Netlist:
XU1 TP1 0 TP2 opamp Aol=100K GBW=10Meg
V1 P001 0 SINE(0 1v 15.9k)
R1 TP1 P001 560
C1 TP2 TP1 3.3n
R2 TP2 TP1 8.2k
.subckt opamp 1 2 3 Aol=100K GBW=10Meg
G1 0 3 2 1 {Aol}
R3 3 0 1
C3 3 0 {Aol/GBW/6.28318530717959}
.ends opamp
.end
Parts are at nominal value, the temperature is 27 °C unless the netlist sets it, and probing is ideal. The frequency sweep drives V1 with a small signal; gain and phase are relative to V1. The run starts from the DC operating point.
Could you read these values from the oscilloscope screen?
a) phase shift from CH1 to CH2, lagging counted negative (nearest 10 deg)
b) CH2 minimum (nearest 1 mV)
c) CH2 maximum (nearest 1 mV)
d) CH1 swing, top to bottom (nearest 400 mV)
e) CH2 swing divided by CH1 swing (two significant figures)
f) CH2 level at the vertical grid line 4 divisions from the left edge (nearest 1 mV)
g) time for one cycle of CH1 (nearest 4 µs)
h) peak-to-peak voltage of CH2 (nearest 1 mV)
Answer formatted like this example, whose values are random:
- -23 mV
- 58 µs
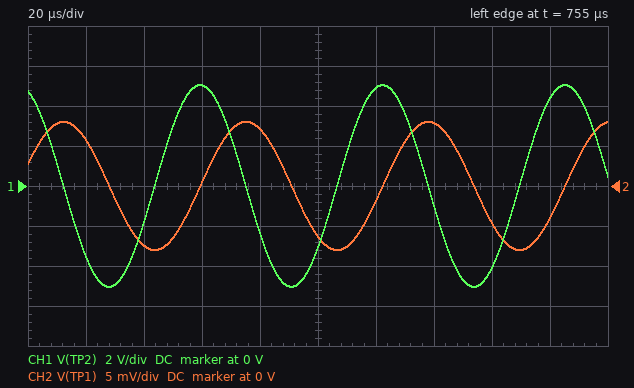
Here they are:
- -90 deg
- -8 mV
- 8 mV
- 10.0 V
- 0.0016
- 7 mV
- 64 µs
- 16 mV
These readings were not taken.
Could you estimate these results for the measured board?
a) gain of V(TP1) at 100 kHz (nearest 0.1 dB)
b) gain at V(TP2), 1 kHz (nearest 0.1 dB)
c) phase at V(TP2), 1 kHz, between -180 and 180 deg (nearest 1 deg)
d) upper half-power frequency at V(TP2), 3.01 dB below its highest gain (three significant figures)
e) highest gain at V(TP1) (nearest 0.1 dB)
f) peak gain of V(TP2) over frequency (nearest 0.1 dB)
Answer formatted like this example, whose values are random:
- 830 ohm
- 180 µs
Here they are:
- -41.4 dB
- 23.2 dB
- 170 deg
- 5.83 kHz
- -41.4 dB
- 23.3 dB
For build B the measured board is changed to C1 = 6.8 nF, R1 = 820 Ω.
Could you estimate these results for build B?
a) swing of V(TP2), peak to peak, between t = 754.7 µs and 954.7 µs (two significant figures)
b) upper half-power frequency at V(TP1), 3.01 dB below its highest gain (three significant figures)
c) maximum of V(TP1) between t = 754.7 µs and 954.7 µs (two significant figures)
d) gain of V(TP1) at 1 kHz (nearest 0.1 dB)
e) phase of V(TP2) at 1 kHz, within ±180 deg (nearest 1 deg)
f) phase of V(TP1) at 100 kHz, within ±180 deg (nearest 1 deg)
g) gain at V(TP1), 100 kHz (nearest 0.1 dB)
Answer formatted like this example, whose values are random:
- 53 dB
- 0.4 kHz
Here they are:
- 3.5 V
- 10.0 MHz
- 2.8 mV
- -60.5 dB
- 161 deg
- 1 deg
- -50.9 dB
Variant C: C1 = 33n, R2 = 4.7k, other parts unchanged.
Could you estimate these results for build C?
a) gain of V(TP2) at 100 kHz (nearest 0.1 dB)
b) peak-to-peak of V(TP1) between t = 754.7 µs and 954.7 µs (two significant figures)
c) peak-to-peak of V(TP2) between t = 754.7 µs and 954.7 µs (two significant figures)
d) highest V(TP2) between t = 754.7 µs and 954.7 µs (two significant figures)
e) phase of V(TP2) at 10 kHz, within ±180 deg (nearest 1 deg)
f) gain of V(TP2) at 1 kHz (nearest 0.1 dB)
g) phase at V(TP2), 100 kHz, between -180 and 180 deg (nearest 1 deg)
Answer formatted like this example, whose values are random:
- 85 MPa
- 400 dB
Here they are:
- -21.3 dB
- 1.7 mV
- 1.1 V
- 540 mV
- 96 deg
- 15.6 dB
- 90 deg
